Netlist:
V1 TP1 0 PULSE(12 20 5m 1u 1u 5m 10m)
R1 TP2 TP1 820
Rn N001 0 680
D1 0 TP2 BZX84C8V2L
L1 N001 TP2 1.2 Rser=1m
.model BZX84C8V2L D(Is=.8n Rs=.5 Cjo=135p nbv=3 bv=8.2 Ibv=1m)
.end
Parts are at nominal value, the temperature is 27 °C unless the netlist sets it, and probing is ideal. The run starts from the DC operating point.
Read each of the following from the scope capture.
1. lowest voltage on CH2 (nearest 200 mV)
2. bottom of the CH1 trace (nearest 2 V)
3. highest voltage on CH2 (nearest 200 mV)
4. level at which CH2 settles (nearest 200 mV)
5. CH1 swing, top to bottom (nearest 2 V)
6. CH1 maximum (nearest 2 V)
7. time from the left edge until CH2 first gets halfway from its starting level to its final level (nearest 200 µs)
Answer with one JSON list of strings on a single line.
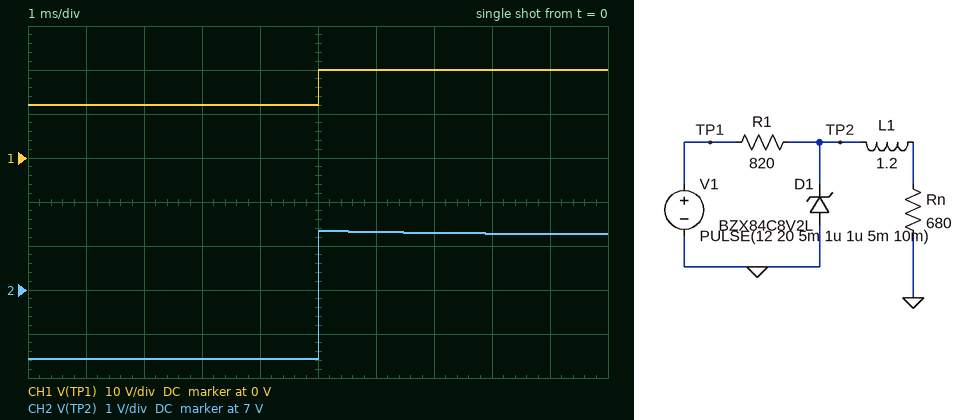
["5.4 V", "12 V", "8.4 V", "8.2 V", "8 V", "20 V", "5.0 ms"]
